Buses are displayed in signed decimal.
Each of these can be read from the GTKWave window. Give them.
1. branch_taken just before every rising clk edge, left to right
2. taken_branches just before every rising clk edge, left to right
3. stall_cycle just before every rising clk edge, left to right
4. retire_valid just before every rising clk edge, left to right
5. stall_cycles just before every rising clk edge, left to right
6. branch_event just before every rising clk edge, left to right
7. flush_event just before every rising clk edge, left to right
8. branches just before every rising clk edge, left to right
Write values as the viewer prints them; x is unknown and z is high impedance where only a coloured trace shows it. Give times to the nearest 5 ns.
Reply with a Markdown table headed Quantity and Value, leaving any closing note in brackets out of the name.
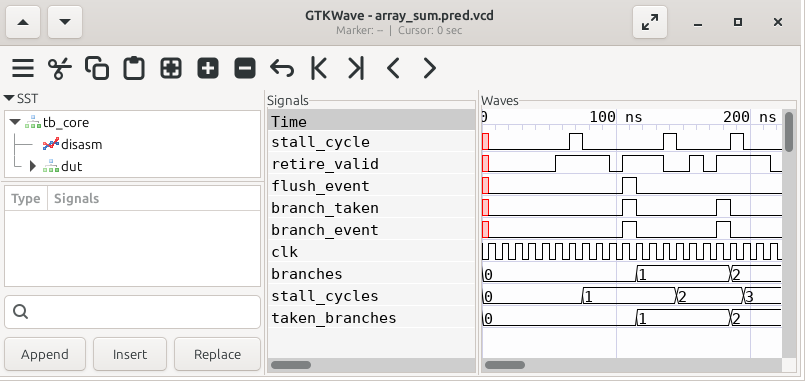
| Quantity | Value |
|---|---|
| branch_taken just before every rising clk edge, left to right | x 0 0 0 0 0 0 0 0 0 0 1 0 0 0 0 0 0 1 0 0 0 |
| taken_branches just before every rising clk edge, left to right | 0, 0, 0, 0, 0, 0, 0, 0, 0, 0, 0, 0, 1, 1, 1, 1, 1, 1, 1, 2, 2, 2 |
| stall_cycle just before every rising clk edge, left to right | x 0 0 0 0 0 0 1 0 0 0 0 0 0 1 0 0 0 0 1 0 0 |
| retire_valid just before every rising clk edge, left to right | x 0 0 0 0 0 1 1 1 1 0 1 1 1 0 0 1 0 1 1 1 1 |
| stall_cycles just before every rising clk edge, left to right | 0, 0, 0, 0, 0, 0, 0, 0, 1, 1, 1, 1, 1, 1, 1, 2, 2, 2, 2, 2, 3, 3 |
| branch_event just before every rising clk edge, left to right | x 0 0 0 0 0 0 0 0 0 0 1 0 0 0 0 0 0 1 0 0 0 |
| flush_event just before every rising clk edge, left to right | x 0 0 0 0 0 0 0 0 0 0 1 0 0 0 0 0 0 0 0 0 0 |
| branches just before every rising clk edge, left to right | 0, 0, 0, 0, 0, 0, 0, 0, 0, 0, 0, 0, 1, 1, 1, 1, 1, 1, 1, 2, 2, 2 |
